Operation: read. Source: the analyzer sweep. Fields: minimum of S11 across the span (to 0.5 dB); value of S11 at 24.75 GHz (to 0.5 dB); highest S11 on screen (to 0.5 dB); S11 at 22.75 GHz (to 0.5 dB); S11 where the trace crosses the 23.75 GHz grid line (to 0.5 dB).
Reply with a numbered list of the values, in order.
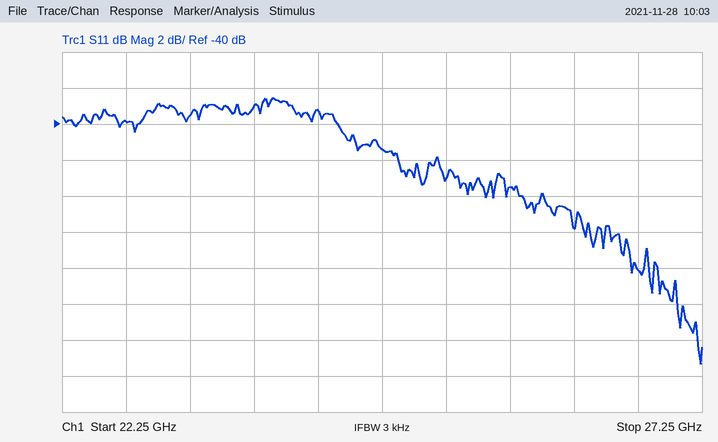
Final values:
1. -53.5 dB
2. -41.5 dB
3. -38.5 dB
4. -40.0 dB
5. -39.0 dB
